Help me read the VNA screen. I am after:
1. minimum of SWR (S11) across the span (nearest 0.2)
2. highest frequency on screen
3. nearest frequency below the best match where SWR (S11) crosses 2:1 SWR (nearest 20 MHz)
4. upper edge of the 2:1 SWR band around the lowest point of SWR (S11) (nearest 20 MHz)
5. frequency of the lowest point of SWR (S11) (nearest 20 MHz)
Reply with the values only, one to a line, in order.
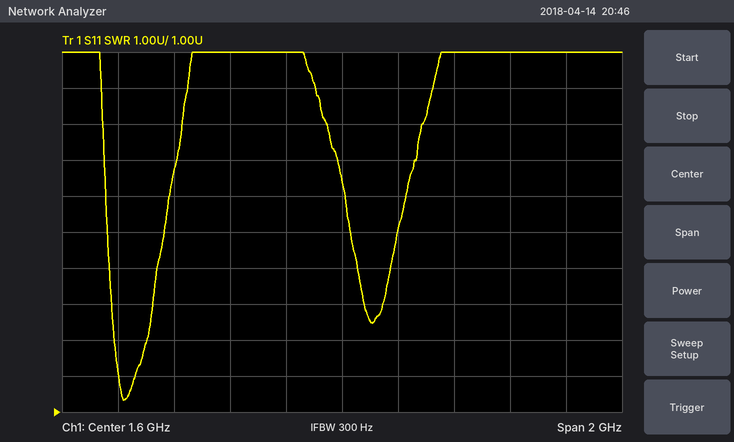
1.4
2.6 GHz
800 MHz
860 MHz
820 MHz
